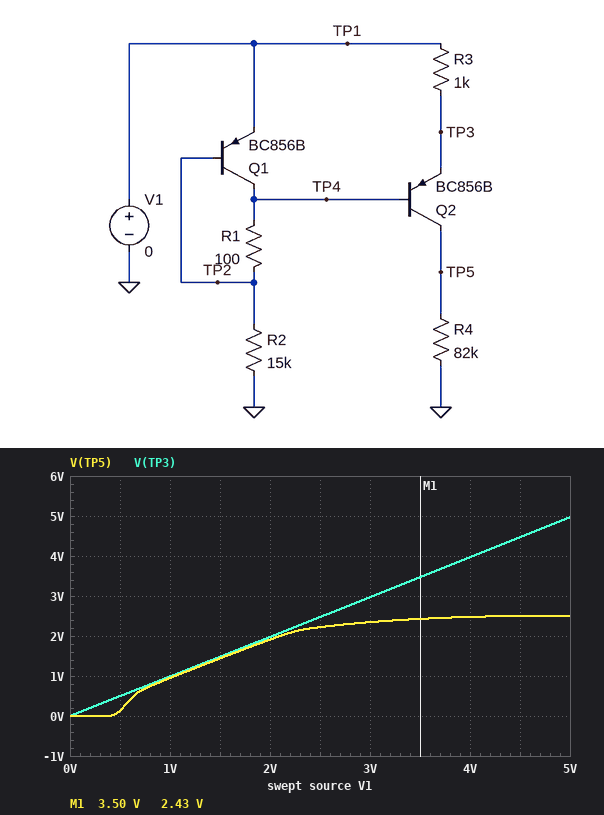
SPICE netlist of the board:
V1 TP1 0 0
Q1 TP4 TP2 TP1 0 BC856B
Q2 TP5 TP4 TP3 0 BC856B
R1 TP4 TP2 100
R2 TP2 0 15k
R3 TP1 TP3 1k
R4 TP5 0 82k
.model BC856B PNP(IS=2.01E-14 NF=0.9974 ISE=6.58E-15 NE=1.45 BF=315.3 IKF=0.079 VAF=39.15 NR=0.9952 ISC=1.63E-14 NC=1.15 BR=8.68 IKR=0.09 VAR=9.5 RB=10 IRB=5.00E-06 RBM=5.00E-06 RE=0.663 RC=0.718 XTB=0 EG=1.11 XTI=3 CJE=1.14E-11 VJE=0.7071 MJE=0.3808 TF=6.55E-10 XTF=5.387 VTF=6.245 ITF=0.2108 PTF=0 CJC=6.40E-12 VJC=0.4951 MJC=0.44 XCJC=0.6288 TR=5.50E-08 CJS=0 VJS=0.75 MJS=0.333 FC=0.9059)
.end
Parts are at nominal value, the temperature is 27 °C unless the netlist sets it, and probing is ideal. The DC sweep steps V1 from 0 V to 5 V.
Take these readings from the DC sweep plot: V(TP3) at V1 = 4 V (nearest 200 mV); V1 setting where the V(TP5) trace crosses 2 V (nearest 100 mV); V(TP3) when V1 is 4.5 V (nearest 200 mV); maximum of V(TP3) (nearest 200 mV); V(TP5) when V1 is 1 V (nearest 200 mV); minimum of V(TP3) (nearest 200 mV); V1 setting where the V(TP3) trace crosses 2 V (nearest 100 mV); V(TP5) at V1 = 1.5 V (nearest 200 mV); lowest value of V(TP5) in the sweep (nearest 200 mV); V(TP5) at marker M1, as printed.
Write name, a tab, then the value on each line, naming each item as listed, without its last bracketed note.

V(TP3) at V1 = 4 V	4.0 V
V1 setting where the V(TP5) trace crosses 2 V	2.1 V
V(TP3) when V1 is 4.5 V	4.4 V
maximum of V(TP3)	5.0 V
V(TP5) when V1 is 1 V	1.0 V
minimum of V(TP3)	0 V
V1 setting where the V(TP3) trace crosses 2 V	2.0 V
V(TP5) at V1 = 1.5 V	1.4 V
lowest value of V(TP5) in the sweep	0 V
V(TP5) at marker M1, as printed	2.43 V
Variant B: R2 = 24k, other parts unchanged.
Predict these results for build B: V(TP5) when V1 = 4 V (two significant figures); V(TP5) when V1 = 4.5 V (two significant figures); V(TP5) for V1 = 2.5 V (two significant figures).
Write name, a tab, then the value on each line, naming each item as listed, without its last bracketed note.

V(TP5) when V1 = 4 V	2.3 V
V(TP5) when V1 = 4.5 V	2.4 V
V(TP5) for V1 = 2.5 V	1.9 V
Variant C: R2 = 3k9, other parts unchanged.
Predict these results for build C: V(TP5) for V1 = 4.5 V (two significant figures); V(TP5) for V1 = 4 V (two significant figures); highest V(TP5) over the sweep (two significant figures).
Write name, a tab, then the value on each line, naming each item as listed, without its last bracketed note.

V(TP5) for V1 = 4.5 V	1.2 V
V(TP5) for V1 = 4 V	1.4 V
highest V(TP5) over the sweep	2.2 V
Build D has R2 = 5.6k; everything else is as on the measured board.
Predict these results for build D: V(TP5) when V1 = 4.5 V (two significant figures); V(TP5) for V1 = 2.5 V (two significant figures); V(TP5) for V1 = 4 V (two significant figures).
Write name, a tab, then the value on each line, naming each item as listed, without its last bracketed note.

V(TP5) when V1 = 4.5 V	1.8 V
V(TP5) for V1 = 2.5 V	2.4 V
V(TP5) for V1 = 4 V	2.0 V
